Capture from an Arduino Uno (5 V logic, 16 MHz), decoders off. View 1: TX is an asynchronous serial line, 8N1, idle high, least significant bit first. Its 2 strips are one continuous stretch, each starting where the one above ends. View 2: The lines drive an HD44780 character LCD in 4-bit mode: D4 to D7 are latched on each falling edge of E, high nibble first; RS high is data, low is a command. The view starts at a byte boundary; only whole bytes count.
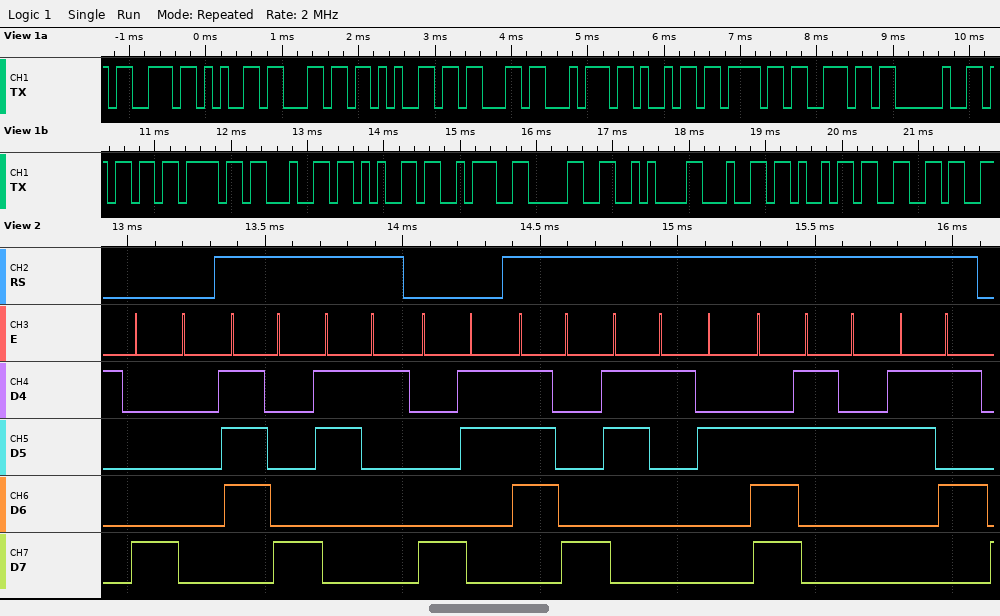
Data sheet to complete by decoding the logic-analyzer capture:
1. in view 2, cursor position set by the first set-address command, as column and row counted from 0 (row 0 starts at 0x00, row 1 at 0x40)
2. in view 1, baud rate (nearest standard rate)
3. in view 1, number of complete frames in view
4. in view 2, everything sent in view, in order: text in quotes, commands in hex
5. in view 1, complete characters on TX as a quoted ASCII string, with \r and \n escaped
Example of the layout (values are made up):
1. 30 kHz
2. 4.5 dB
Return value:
1. column 0, row 0
2. 9600 baud
3. 20
4. 0x80 "x1" 0x83 "x1.25"
5. "selection mode:0\ndif"
